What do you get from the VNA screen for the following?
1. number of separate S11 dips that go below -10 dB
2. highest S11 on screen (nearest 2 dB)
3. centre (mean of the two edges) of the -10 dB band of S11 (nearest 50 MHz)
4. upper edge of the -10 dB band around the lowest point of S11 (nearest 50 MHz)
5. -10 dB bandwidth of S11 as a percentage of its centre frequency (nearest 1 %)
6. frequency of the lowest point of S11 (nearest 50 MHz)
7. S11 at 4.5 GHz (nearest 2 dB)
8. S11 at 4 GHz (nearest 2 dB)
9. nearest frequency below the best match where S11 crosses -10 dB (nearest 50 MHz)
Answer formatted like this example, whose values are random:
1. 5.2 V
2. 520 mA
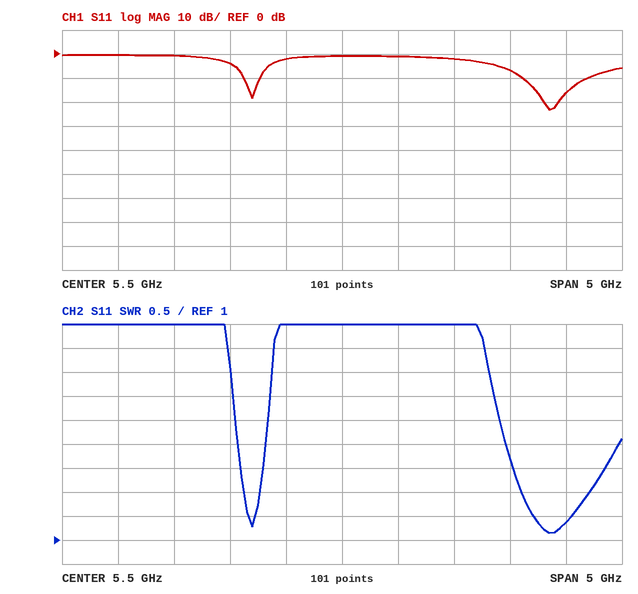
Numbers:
1. 2
2. 0 dB
3. 7.40 GHz
4. 7.70 GHz
5. 8 %
6. 7.35 GHz
7. -4 dB
8. 0 dB
9. 7.10 GHz
